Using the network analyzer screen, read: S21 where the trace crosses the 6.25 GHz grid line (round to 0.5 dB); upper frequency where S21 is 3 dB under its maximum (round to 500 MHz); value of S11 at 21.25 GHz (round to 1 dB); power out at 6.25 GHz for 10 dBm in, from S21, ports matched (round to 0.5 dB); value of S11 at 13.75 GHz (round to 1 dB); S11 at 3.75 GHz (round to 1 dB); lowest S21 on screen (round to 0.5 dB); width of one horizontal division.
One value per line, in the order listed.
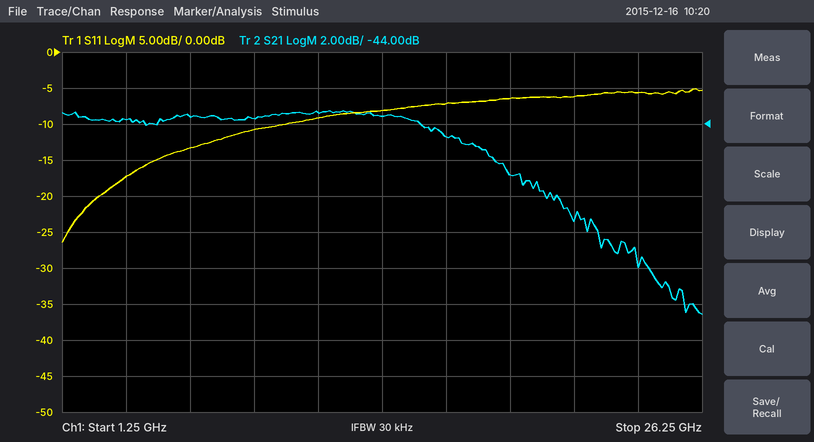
-43.5 dB
18.5 GHz
-6 dB
-33.5 dBm
-8 dB
-17 dB
-54.5 dB
2.5 GHz
